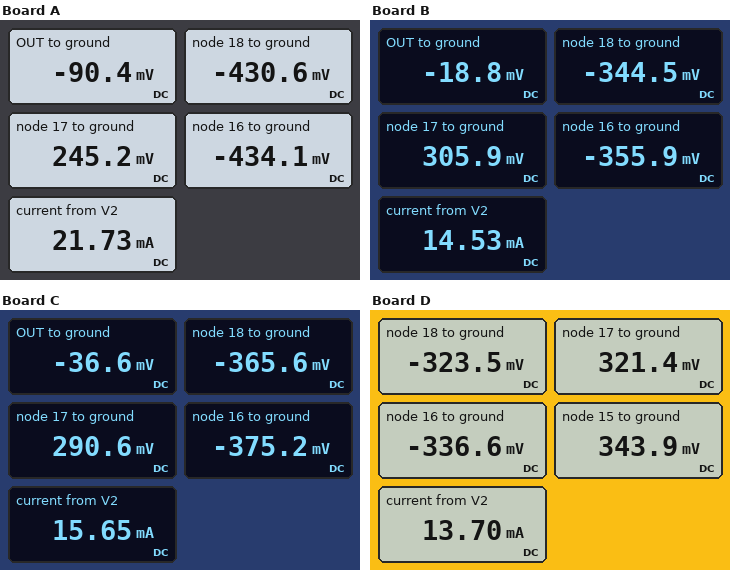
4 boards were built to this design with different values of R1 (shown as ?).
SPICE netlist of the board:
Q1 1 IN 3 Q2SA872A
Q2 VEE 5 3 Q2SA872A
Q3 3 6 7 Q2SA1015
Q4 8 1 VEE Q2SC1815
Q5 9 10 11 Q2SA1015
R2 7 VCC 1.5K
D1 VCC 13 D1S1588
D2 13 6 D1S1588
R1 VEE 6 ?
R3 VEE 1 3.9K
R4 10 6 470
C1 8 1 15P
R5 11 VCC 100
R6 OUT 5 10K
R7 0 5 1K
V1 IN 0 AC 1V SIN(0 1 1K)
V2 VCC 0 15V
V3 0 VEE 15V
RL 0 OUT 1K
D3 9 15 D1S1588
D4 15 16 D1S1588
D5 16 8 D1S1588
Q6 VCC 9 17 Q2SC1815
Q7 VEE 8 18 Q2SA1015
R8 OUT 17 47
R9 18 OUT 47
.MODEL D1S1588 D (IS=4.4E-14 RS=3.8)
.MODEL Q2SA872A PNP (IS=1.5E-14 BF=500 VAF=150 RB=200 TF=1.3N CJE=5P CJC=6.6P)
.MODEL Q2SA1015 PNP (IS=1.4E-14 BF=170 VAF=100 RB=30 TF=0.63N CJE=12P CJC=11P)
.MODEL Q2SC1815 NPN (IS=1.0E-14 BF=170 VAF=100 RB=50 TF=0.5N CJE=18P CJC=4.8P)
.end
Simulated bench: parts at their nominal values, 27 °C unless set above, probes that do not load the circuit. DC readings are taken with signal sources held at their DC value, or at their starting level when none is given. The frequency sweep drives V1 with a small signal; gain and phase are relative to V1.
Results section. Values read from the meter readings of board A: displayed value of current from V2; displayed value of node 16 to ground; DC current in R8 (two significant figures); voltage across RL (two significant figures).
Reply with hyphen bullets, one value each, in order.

- 21.73 mA
- -434.1 mV
- 7.1 mA
- 90 mV
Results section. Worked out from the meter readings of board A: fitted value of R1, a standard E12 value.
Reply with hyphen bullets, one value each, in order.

- 3.9 kΩ
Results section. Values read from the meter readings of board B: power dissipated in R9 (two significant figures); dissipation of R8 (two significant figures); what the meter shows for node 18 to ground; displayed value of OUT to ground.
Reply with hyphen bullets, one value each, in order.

- 2.3 mW
- 2.2 mW
- -344.5 mV
- -18.8 mV
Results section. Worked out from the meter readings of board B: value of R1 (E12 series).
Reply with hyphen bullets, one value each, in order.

- 18 kΩ
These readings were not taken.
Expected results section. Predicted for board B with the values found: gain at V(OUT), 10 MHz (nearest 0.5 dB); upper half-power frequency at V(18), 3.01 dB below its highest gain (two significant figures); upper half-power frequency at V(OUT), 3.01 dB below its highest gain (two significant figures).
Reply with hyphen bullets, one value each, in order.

- 10.5 dB
- 4.9 MHz
- 4.9 MHz
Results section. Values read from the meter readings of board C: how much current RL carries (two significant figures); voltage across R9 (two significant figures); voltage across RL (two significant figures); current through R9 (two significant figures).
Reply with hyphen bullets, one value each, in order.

- 37 µA
- 330 mV
- 37 mV
- 7.0 mA
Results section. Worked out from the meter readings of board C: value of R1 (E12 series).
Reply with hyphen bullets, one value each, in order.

- 12 kΩ
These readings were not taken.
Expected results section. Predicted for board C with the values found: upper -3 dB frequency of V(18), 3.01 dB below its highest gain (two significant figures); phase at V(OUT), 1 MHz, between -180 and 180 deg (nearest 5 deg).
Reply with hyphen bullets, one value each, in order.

- 5.2 MHz
- -15 deg
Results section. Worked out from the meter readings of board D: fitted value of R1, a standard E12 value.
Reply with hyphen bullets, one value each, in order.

- 27 kΩ
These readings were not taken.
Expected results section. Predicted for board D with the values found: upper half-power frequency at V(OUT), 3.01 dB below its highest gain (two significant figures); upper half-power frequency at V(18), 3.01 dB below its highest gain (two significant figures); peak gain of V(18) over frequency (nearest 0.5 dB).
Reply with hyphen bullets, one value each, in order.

- 4.7 MHz
- 4.7 MHz
- 21.0 dB
